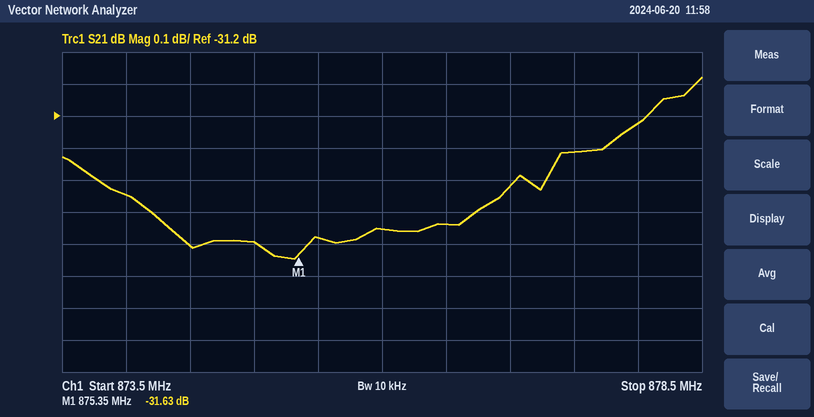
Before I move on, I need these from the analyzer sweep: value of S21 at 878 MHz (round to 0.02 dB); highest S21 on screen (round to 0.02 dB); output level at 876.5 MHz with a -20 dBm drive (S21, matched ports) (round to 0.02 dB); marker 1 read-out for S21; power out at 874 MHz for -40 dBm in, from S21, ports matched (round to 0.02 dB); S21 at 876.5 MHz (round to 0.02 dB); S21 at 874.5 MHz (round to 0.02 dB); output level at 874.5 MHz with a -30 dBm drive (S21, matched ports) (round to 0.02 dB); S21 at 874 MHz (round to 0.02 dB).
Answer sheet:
-31.22 dB
-31.08 dB
-51.54 dBm
-31.63 dB
-71.44 dBm
-31.54 dB
-31.60 dB
-61.60 dBm
-31.44 dB
